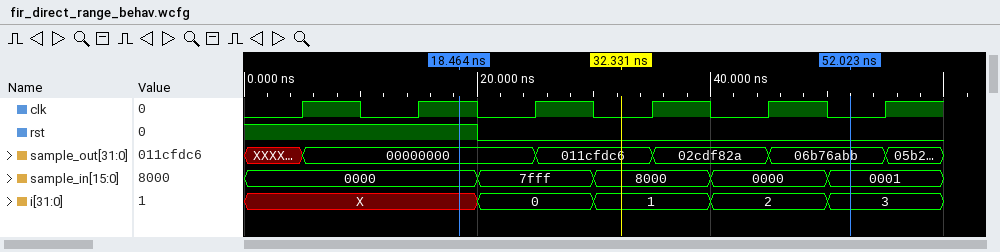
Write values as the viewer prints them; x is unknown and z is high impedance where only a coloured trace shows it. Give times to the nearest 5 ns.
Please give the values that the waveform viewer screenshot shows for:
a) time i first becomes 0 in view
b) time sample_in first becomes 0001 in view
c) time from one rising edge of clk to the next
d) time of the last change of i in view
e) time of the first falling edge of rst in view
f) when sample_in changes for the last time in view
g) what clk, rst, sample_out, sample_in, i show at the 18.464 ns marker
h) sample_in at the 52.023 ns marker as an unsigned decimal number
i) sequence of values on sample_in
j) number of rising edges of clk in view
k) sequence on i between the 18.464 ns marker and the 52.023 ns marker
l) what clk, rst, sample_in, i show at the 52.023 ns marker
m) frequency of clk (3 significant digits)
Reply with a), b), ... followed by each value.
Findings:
a) 20 ns
b) 50 ns
c) 10 ns
d) 50 ns
e) 20 ns
f) 50 ns
g) clk=1, rst=1, sample_out=00000000, sample_in=0000, i=X
h) 1
i) 0000, 7fff, 8000, 0000, 0001
j) 6
k) X, 0, 1, 2, 3
l) clk=0, rst=0, sample_in=0001, i=3
m) 100 MHz
